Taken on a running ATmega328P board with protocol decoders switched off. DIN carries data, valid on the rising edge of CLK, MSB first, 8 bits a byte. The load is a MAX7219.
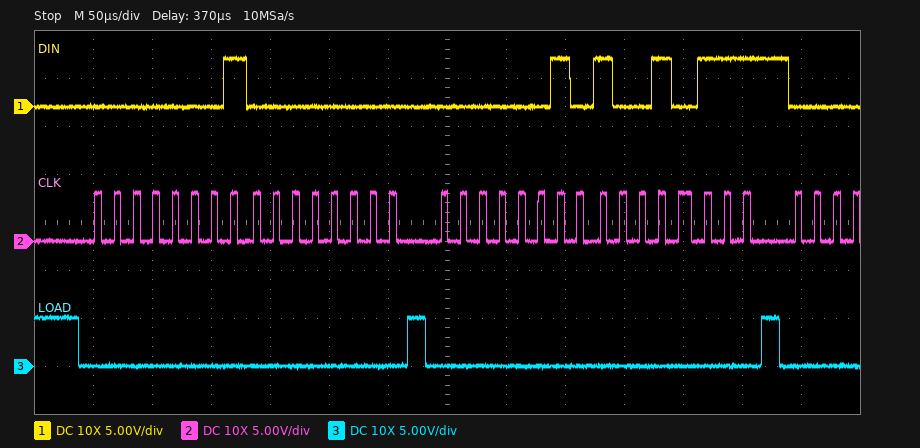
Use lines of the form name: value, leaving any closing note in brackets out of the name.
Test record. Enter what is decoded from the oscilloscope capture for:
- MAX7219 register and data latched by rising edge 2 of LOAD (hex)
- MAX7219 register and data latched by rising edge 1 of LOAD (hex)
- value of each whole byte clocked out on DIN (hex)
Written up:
MAX7219 register and data latched by rising edge 2 of LOAD: register 0x2, data 0x97
MAX7219 register and data latched by rising edge 1 of LOAD: register 0x1, data 0x00
value of each whole byte clocked out on DIN: 01 00 02 97
